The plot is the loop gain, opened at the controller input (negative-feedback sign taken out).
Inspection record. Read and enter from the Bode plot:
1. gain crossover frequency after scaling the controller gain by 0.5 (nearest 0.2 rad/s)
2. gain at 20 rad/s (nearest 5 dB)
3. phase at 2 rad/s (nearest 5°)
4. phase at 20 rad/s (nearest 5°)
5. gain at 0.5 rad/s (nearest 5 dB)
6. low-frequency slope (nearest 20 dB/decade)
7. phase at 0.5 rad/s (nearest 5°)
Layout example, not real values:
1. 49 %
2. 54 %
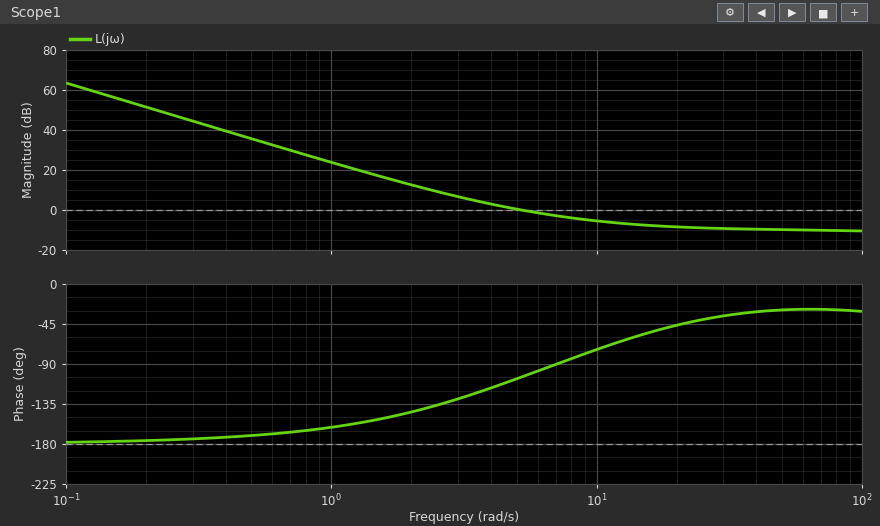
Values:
1. 3.2 rad/s
2. -10 dB
3. -145°
4. -45°
5. 35 dB
6. -40 dB/decade
7. -170°
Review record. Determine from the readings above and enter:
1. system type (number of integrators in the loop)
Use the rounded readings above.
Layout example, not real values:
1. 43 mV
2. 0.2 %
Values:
1. 2
